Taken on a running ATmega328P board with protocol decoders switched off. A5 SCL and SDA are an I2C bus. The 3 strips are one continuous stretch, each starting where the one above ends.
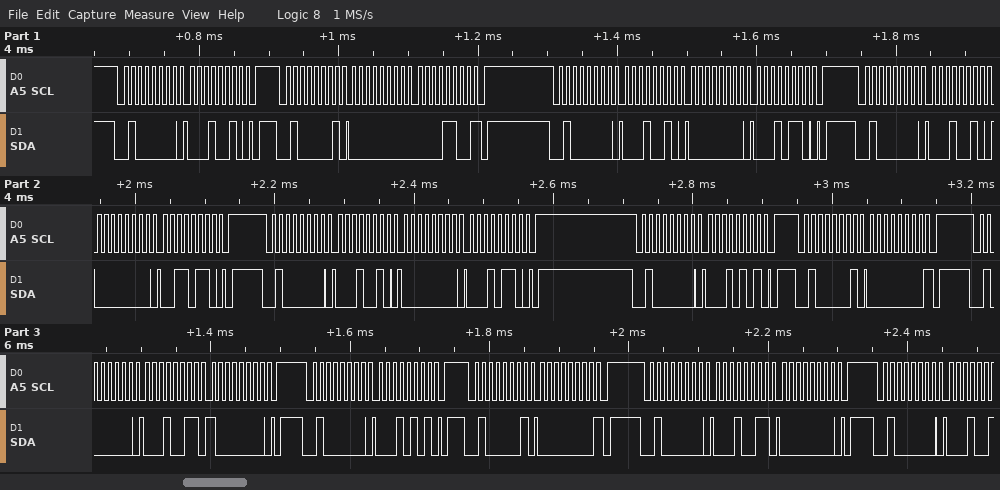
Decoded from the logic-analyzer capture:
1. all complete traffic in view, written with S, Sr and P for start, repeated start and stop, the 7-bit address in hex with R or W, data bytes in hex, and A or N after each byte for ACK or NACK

S 20W A 12 A P S 20R A 00 A 0C N P S 20W A 12 A 00 A 16 A P S 20W A 12 A 00 A 36 A P S 20W A 12 A 00 A 16 A P S 20W A 15 A P S 20R A 00 N P S 20W A 13 A 80 A P S 20W A 15 A P S 20R A 00 N P S 20W A 13 A 00 A P S 20W A
